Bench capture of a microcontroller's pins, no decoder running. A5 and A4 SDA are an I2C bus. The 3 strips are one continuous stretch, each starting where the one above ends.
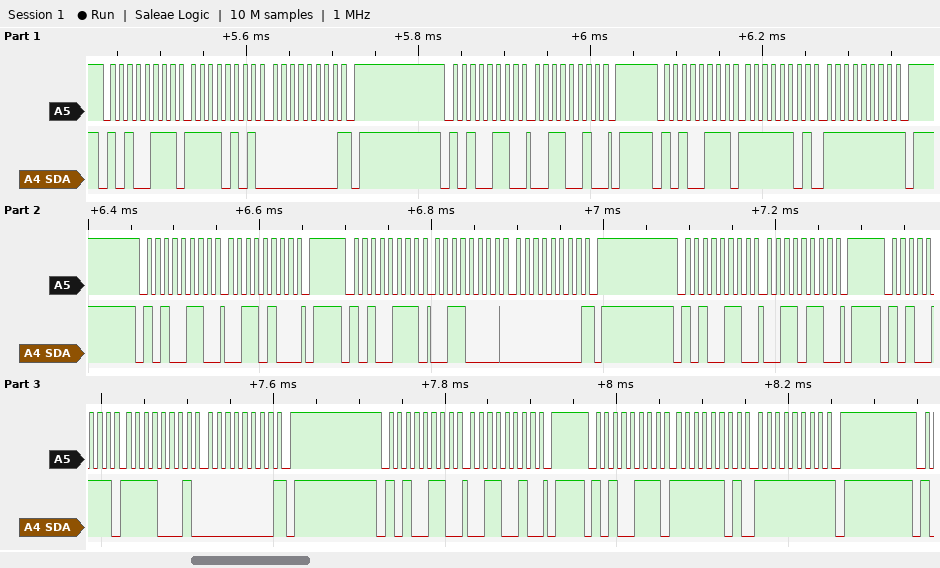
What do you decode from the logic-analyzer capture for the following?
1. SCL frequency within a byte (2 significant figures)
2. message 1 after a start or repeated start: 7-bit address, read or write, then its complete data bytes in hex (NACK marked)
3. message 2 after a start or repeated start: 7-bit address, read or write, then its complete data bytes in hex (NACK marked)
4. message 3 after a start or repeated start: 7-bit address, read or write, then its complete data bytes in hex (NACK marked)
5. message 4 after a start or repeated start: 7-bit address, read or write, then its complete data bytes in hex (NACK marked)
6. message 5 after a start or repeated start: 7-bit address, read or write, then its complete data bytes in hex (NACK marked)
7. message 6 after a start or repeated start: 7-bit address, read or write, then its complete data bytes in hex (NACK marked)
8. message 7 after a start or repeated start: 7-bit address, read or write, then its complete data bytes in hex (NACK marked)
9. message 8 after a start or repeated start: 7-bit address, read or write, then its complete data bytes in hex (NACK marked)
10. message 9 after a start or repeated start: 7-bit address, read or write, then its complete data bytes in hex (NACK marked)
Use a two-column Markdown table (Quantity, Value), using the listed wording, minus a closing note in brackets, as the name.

| Quantity | Value |
|---|---|
| SCL frequency within a byte | 100 kHz |
| message 1 after a start or repeated start: 7-bit address, read or write, then its complete data bytes in hex | 0x53 read: F5 00 NACK |
| message 2 after a start or repeated start: 7-bit address, read or write, then its complete data bytes in hex | 0x53 write: 32 |
| message 3 after a start or repeated start: 7-bit address, read or write, then its complete data bytes in hex | 0x53 read: FD FF NACK |
| message 4 after a start or repeated start: 7-bit address, read or write, then its complete data bytes in hex | 0x53 write: 34 |
| message 5 after a start or repeated start: 7-bit address, read or write, then its complete data bytes in hex | 0x53 read: 30 00 NACK |
| message 6 after a start or repeated start: 7-bit address, read or write, then its complete data bytes in hex | 0x53 write: 36 |
| message 7 after a start or repeated start: 7-bit address, read or write, then its complete data bytes in hex | 0x53 read: F1 00 NACK |
| message 8 after a start or repeated start: 7-bit address, read or write, then its complete data bytes in hex | 0x53 write: 32 |
| message 9 after a start or repeated start: 7-bit address, read or write, then its complete data bytes in hex | 0x53 read: FD FF NACK |
